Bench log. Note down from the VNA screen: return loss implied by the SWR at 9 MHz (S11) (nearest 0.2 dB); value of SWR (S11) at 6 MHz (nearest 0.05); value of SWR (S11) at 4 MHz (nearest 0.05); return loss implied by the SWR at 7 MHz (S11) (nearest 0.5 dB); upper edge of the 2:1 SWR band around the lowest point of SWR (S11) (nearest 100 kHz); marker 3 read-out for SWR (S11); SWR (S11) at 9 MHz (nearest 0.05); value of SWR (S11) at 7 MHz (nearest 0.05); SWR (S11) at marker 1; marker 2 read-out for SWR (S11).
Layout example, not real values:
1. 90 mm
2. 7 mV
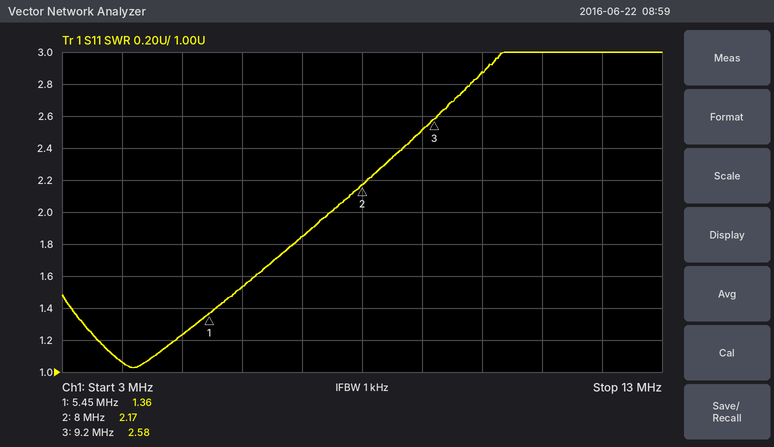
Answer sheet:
1. 7.4 dB
2. 1.55
3. 1.05
4. 10.5 dB
5. 7.5 MHz
6. 2.58
7. 2.50
8. 1.85
9. 1.36
10. 2.17
